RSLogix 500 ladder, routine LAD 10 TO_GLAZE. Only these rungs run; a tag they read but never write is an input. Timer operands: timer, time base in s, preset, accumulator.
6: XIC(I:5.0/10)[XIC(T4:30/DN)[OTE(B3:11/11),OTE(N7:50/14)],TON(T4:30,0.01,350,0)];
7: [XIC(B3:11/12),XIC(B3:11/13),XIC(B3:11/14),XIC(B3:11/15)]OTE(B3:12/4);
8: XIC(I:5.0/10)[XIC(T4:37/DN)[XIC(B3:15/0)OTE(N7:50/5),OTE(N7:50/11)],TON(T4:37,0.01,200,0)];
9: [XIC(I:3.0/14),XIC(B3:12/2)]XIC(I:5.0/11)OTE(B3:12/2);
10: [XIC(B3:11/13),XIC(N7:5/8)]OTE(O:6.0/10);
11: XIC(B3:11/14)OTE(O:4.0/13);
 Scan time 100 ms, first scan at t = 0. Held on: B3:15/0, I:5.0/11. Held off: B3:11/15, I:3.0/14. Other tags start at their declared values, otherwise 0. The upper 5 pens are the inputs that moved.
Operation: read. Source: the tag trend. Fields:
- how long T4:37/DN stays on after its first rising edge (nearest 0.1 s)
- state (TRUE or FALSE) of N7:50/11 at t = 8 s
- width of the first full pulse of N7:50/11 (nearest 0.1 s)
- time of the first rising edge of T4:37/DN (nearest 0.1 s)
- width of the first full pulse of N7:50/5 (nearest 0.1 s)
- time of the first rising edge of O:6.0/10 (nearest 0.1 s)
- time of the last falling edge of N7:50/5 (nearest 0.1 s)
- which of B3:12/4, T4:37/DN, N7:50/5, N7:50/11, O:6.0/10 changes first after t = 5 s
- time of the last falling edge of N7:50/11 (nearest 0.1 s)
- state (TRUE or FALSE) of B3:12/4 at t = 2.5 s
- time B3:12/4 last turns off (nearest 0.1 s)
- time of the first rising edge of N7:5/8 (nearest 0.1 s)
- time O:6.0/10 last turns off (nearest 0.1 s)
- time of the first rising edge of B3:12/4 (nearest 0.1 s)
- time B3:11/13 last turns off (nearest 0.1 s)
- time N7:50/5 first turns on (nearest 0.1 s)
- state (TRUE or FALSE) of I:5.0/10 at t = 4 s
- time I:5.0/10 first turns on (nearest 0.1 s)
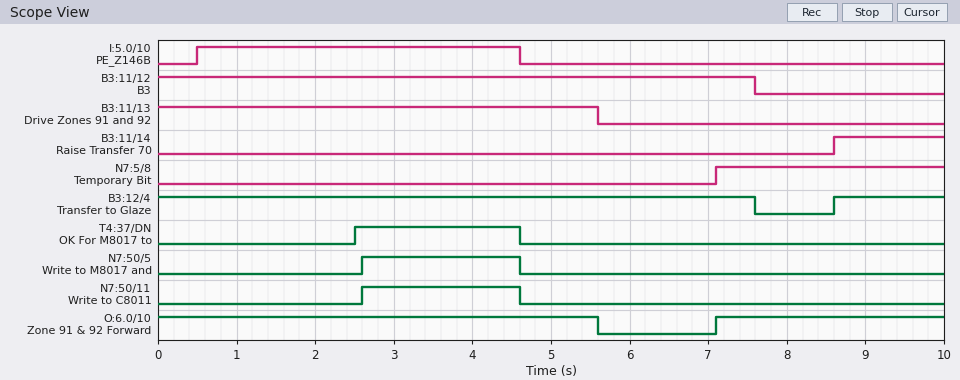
2.1 s
FALSE
2.0 s
2.5 s
2.0 s
7.1 s
4.6 s
O:6.0/10
4.6 s
TRUE
7.6 s
7.1 s
5.6 s
8.6 s
5.6 s
2.6 s
TRUE
0.5 s
